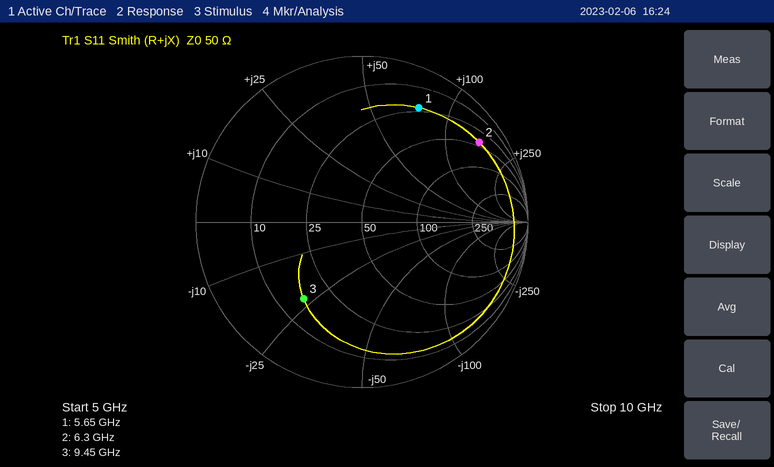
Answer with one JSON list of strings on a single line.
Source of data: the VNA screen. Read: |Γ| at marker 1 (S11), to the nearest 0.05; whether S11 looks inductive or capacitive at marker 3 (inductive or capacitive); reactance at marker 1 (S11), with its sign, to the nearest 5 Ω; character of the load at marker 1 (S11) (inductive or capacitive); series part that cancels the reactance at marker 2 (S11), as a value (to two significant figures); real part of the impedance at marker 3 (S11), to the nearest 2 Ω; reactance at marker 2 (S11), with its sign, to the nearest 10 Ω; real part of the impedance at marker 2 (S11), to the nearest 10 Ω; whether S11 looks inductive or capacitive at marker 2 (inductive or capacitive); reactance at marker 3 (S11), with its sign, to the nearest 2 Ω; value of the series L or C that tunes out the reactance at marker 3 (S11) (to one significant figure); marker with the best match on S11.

["0.75", "capacitive", "+75 Ω", "inductive", "170 fF", "16 Ω", "+150 Ω", "40 Ω", "inductive", "-22 Ω", "400 pH", "marker 3"]
